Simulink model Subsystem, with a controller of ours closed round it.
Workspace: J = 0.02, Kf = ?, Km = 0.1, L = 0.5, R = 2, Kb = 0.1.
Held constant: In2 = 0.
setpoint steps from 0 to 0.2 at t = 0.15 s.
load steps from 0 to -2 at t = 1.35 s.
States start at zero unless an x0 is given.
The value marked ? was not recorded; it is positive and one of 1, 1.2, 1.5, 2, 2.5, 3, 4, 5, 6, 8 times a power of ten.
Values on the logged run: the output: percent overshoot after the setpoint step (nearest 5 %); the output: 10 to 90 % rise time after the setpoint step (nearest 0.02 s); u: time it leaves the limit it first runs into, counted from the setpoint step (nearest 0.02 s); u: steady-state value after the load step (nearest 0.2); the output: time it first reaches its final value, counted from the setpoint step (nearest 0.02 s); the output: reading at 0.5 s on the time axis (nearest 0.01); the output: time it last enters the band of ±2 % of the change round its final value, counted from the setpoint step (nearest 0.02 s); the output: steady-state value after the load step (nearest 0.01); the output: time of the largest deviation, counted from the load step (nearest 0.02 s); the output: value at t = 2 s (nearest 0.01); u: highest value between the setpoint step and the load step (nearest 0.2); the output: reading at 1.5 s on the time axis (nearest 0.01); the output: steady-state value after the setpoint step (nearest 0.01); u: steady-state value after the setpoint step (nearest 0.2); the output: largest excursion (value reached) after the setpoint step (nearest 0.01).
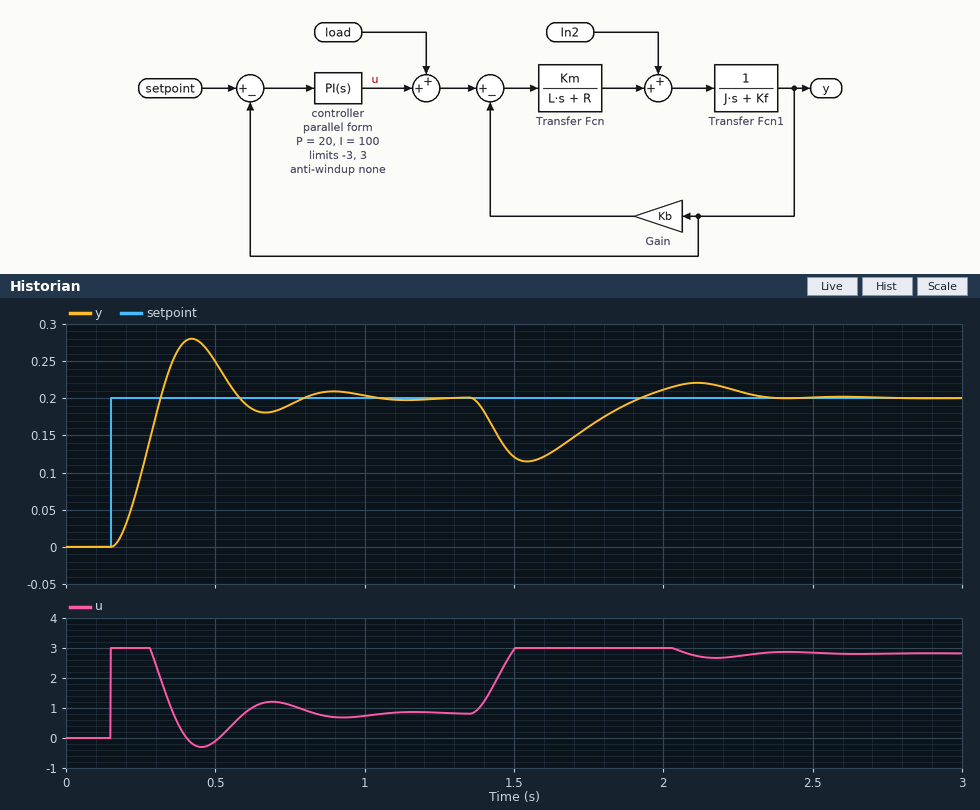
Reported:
40 %
0.12 s
0.14 s
2.8
0.16 s
0.25
0.84 s
0.20
0.20 s
0.21
3.0
0.12
0.20
0.8
0.28
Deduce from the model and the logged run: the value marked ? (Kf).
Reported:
0.2
